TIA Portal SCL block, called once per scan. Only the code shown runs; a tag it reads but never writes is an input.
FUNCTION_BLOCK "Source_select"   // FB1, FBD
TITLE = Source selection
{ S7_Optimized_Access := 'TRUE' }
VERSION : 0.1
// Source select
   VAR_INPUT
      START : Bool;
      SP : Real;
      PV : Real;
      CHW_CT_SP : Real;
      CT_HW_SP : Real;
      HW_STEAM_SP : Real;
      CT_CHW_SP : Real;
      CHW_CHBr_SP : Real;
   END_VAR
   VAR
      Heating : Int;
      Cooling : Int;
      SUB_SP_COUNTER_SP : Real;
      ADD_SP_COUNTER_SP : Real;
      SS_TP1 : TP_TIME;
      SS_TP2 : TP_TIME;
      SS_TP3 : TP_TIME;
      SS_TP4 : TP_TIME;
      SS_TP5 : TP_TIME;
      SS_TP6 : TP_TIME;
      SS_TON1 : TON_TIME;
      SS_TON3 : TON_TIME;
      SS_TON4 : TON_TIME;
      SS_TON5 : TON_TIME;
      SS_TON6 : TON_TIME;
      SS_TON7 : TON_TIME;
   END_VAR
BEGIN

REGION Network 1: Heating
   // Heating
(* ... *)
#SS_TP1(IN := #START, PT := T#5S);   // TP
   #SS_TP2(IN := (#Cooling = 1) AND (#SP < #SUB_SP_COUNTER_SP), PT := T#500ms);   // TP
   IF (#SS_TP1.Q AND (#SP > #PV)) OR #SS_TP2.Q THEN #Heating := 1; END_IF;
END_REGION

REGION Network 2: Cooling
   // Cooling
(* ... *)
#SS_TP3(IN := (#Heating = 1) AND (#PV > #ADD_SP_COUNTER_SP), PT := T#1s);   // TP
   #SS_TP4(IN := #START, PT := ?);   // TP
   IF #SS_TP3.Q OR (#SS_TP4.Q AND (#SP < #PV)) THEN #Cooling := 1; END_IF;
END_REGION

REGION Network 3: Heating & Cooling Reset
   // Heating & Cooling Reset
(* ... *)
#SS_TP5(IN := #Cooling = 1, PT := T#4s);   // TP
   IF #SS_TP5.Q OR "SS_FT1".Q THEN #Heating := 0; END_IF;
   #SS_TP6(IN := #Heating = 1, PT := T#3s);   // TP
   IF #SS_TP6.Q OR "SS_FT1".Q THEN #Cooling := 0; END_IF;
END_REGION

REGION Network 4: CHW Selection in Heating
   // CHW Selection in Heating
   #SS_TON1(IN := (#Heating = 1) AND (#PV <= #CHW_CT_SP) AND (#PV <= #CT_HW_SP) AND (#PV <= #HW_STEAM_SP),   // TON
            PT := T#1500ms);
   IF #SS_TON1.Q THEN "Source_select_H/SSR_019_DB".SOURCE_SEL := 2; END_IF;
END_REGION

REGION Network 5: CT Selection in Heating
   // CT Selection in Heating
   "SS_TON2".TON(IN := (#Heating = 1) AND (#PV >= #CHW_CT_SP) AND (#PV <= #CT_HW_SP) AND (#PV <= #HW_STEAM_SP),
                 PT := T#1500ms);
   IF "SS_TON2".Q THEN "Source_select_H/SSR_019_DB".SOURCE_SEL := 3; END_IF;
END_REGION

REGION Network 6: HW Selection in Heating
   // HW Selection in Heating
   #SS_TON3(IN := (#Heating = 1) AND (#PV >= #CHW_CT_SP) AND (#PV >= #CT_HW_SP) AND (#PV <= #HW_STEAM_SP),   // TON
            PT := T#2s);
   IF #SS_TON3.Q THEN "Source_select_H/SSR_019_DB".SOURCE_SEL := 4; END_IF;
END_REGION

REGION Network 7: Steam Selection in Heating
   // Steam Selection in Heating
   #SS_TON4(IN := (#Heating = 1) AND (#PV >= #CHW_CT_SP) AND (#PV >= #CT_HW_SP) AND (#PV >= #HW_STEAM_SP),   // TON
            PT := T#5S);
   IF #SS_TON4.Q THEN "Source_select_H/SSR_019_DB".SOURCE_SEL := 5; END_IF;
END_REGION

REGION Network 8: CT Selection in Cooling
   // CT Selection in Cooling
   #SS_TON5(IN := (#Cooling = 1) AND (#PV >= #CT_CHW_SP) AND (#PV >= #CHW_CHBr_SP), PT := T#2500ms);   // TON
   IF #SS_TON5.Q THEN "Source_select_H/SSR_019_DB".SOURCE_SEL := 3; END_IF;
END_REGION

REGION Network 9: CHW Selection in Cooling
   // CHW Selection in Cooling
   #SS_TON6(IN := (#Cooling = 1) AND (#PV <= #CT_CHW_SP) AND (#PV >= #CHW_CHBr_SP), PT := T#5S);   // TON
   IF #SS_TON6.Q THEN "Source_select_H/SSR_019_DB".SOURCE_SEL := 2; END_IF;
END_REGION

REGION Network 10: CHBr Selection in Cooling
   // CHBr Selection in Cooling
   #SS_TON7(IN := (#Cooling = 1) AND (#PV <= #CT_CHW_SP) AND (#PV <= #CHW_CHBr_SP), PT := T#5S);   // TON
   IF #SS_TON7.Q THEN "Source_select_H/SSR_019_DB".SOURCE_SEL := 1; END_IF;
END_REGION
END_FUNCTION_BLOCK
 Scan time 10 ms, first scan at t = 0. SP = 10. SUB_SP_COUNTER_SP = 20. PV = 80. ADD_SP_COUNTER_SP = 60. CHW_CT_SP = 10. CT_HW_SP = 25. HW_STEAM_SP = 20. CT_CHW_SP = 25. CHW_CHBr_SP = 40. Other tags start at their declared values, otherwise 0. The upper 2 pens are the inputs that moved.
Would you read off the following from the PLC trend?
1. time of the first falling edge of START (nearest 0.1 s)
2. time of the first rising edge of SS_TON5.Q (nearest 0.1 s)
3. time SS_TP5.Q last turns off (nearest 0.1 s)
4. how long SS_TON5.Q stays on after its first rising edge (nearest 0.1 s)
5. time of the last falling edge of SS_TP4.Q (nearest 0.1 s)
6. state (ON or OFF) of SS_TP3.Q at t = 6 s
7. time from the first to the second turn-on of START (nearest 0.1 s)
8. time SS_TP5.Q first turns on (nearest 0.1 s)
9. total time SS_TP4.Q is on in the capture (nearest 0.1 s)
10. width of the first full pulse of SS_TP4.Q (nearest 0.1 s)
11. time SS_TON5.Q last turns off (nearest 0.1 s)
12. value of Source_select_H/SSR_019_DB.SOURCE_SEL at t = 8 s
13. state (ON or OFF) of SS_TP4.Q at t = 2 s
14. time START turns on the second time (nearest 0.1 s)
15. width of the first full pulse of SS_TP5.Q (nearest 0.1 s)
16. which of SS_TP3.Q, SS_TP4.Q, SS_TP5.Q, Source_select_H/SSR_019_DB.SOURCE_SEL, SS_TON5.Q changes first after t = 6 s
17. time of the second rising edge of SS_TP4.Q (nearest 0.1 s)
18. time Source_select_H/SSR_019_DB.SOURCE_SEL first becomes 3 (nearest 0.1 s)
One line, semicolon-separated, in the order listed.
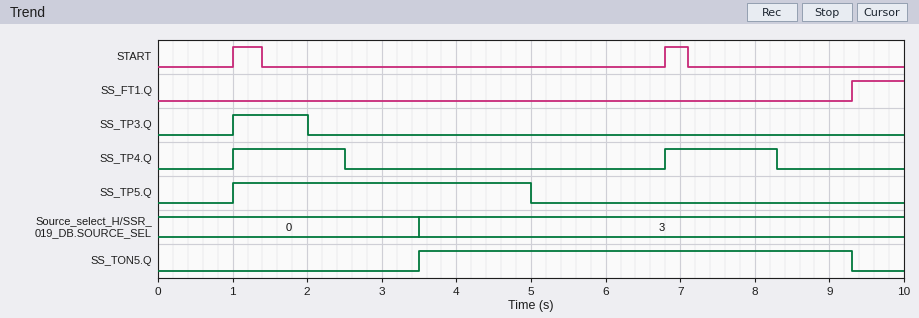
1.4 s; 3.5 s; 5.0 s; 5.8 s; 8.3 s; OFF; 5.8 s; 1.0 s; 3.0 s; 1.5 s; 9.3 s; 3; ON; 6.8 s; 4.0 s; SS_TP4.Q; 6.8 s; 3.5 s
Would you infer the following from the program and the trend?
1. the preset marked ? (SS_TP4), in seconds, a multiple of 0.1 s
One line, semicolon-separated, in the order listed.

1.5 s
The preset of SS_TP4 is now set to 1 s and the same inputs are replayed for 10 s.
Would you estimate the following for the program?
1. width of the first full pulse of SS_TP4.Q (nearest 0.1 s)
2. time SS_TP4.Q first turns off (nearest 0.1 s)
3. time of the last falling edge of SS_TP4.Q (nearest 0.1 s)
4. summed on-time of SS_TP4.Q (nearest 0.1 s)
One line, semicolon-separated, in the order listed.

1.0 s; 2.0 s; 7.8 s; 2.0 s
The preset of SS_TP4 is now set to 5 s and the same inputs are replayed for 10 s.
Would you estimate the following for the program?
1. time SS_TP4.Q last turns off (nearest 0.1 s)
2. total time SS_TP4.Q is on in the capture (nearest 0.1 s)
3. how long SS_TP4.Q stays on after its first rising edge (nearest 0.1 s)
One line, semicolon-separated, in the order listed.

6.0 s; 8.2 s; 5.0 s
